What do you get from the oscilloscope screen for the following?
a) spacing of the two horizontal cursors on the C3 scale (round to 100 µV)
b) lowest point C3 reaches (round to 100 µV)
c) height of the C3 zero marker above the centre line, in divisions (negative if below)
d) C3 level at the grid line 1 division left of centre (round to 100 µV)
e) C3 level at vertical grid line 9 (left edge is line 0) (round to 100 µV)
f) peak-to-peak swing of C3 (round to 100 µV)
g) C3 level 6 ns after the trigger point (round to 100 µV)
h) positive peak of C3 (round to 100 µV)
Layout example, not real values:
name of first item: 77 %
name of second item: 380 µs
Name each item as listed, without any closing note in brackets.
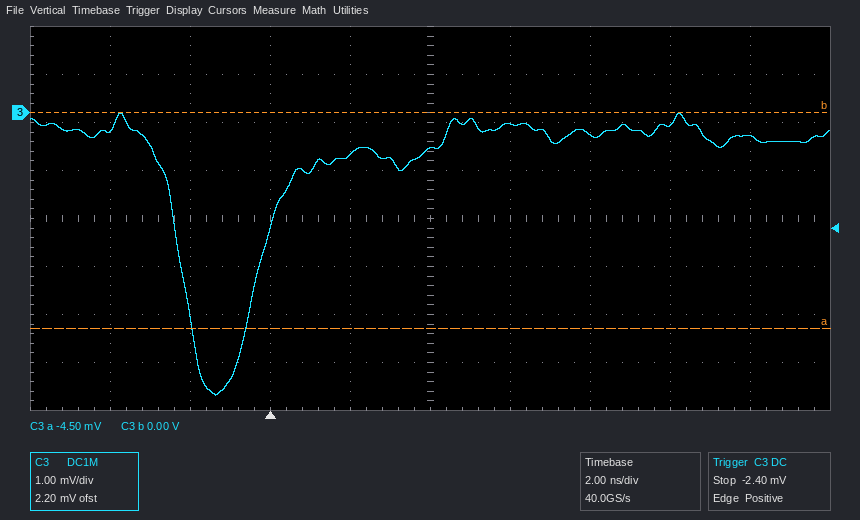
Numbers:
spacing of the two horizontal cursors on the C3 scale: 4.5 mV
lowest point C3 reaches: -5.9 mV
height of the C3 zero marker above the centre line, in divisions: +2.2 div
C3 level at the grid line 1 division left of centre: -900 µV
C3 level at vertical grid line 9 (left edge is line 0): -500 µV
peak-to-peak swing of C3: 5.9 mV
C3 level 6 ns after the trigger point: -200 µV
positive peak of C3: 0.0 mV
